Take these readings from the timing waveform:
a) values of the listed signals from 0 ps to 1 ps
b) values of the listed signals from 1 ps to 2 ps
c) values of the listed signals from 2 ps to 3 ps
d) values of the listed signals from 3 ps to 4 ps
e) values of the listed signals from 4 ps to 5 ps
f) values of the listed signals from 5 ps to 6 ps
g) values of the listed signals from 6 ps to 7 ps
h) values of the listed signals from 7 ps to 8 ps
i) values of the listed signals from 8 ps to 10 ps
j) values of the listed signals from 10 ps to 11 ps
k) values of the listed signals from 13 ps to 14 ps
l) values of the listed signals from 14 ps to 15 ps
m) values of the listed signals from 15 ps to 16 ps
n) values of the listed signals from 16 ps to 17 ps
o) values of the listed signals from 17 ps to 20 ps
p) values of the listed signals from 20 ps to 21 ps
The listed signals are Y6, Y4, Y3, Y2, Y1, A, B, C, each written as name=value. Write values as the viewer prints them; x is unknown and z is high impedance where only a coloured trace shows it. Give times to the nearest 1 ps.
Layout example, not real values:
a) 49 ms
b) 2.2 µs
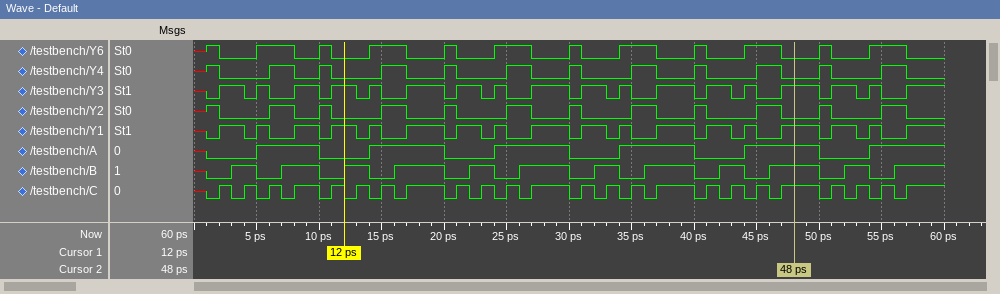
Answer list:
a) Y6=x, Y4=x, Y3=x, Y2=x, Y1=x, A=x, B=x, C=x
b) Y6=1, Y4=1, Y3=0, Y2=1, Y1=0, A=0, B=0, C=0
c) Y6=0, Y4=0, Y3=1, Y2=0, Y1=1, A=0, B=0, C=1
d) Y6=0, Y4=0, Y3=1, Y2=0, Y1=1, A=0, B=1, C=0
e) Y6=0, Y4=0, Y3=0, Y2=0, Y1=0, A=0, B=1, C=1
f) Y6=1, Y4=0, Y3=1, Y2=0, Y1=1, A=1, B=0, C=0
g) Y6=1, Y4=1, Y3=0, Y2=1, Y1=0, A=1, B=0, C=1
h) Y6=1, Y4=1, Y3=0, Y2=1, Y1=0, A=1, B=1, C=0
i) Y6=0, Y4=0, Y3=1, Y2=0, Y1=1, A=1, B=1, C=1
j) Y6=1, Y4=1, Y3=0, Y2=1, Y1=0, A=0, B=0, C=0
k) Y6=0, Y4=0, Y3=0, Y2=0, Y1=0, A=0, B=1, C=1
l) Y6=1, Y4=0, Y3=1, Y2=0, Y1=1, A=1, B=0, C=0
m) Y6=1, Y4=1, Y3=0, Y2=1, Y1=0, A=1, B=0, C=1
n) Y6=1, Y4=1, Y3=0, Y2=1, Y1=0, A=1, B=1, C=0
o) Y6=0, Y4=0, Y3=1, Y2=0, Y1=1, A=1, B=1, C=1
p) Y6=1, Y4=1, Y3=0, Y2=1, Y1=0, A=0, B=0, C=0
